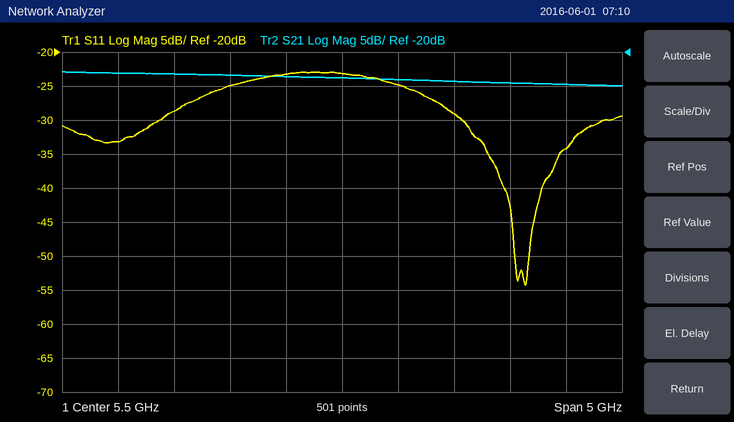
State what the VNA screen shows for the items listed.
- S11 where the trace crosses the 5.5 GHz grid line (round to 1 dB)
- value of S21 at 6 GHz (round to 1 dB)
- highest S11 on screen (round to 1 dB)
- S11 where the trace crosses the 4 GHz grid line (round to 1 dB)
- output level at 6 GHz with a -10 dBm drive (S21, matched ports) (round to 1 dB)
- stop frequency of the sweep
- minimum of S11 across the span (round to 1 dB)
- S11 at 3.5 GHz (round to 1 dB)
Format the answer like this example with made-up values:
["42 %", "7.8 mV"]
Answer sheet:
["-23 dB", "-24 dB", "-23 dB", "-29 dB", "-34 dBm", "8 GHz", "-54 dB", "-33 dB"]
